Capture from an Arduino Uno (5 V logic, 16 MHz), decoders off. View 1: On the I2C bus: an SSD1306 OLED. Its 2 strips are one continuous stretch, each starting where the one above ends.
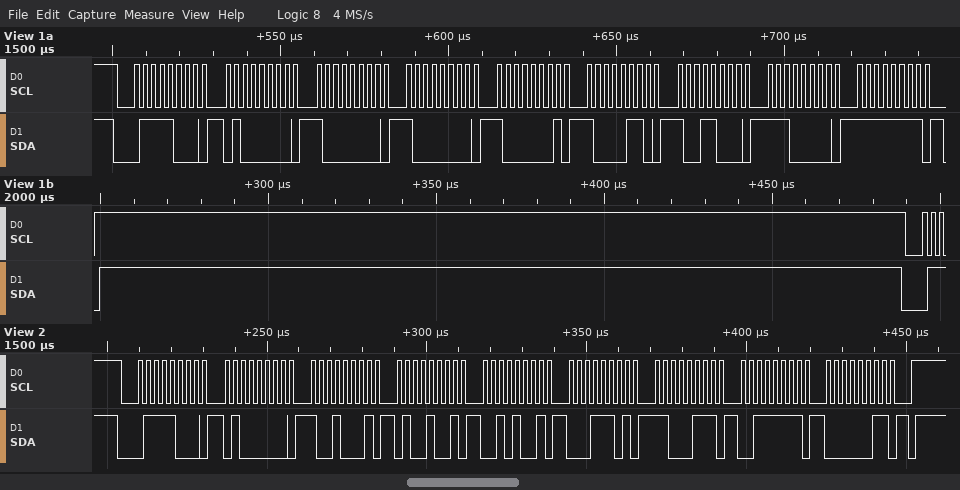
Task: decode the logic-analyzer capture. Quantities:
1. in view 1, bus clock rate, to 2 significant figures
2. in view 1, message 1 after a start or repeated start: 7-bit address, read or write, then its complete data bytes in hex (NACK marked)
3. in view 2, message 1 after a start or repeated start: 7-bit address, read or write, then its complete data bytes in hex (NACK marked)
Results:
400 kHz
0x3C write: 40 80 80 81 86 98 E0 FF
0x3C write: 40 91 49 29 1D C7 3F 03
